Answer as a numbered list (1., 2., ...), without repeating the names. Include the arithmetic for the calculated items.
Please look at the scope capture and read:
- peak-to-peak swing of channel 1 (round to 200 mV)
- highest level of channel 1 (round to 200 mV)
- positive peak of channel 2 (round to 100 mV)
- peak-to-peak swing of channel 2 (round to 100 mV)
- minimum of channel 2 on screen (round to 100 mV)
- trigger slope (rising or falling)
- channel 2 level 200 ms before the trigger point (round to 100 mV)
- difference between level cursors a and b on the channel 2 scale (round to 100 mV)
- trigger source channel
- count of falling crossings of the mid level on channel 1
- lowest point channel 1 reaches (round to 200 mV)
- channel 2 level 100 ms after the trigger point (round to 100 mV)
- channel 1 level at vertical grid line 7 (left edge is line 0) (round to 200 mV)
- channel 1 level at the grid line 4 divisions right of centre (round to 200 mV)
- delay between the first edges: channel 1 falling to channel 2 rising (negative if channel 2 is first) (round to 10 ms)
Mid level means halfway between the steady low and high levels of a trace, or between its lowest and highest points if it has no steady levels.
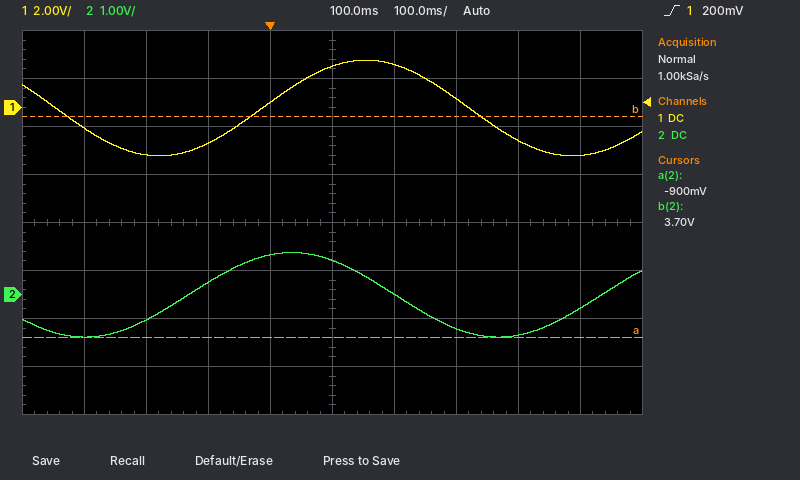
1. 2.0 V − (-2.0 V) = 4.0 V
2. 2.0 V
3. 900 mV
4. 900 mV − (-900 mV) = 1.8 V
5. -900 mV
6. rising
7. -500 mV
8. 4.6 V
9. channel 1
10. 2
11. -2.0 V
12. 700 mV
13. 400 mV
14. -2.0 V
15. +210 ms
